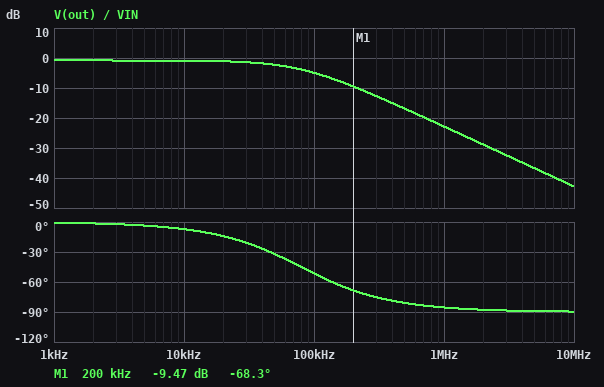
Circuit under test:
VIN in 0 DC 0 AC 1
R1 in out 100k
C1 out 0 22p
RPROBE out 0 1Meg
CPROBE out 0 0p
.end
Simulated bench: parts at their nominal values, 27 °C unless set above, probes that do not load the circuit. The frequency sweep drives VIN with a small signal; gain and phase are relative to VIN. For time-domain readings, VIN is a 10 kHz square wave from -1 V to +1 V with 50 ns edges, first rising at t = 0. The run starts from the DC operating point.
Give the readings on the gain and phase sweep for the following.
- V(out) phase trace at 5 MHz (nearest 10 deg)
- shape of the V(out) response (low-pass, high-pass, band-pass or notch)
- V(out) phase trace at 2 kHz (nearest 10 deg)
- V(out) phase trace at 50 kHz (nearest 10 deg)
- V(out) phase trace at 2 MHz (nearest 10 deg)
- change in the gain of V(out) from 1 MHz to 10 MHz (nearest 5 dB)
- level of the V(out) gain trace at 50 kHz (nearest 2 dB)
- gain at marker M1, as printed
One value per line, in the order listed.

-90 deg
low-pass
0 deg
-30 deg
-90 deg
-20 dB
-2 dB
-9.47 dB
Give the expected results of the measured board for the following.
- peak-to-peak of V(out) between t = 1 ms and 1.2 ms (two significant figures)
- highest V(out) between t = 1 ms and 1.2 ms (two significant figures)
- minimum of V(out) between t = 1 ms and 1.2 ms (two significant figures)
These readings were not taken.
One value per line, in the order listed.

1.8 V
910 mV
-910 mV
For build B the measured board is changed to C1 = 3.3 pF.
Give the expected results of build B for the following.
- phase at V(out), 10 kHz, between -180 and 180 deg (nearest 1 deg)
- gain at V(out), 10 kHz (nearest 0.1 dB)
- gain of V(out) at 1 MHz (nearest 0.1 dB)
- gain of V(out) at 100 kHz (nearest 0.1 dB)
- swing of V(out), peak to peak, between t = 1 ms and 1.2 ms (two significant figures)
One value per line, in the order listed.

-1 deg
-0.8 dB
-7.4 dB
-1.0 dB
1.8 V
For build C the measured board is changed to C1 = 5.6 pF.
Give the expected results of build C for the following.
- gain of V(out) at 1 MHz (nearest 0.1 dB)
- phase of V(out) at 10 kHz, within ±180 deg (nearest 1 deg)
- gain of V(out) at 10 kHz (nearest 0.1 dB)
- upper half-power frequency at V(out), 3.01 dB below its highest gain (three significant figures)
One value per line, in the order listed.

-11.3 dB
-2 deg
-0.8 dB
313 kHz
